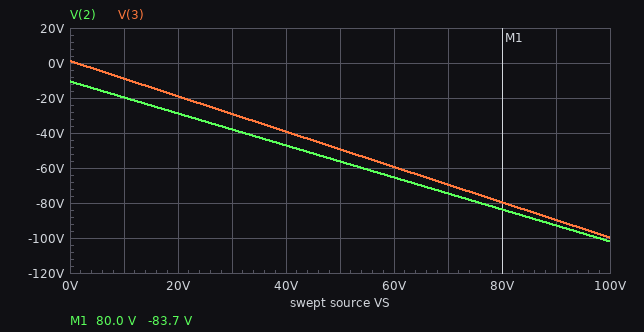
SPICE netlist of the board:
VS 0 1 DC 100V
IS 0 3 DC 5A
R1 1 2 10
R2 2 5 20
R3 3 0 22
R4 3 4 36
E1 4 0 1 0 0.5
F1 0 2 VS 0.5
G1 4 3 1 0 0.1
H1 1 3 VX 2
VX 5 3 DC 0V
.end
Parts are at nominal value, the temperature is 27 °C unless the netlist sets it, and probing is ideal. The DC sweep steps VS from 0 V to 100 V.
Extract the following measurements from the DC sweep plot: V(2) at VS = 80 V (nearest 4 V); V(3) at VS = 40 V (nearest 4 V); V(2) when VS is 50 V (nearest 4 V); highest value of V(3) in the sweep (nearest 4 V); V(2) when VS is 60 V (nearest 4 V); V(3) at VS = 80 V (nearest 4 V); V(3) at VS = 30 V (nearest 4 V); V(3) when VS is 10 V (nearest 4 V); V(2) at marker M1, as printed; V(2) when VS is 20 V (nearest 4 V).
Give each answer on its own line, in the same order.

-84 V
-40 V
-56 V
0 V
-64 V
-80 V
-28 V
-8 V
-83.7 V
-28 V
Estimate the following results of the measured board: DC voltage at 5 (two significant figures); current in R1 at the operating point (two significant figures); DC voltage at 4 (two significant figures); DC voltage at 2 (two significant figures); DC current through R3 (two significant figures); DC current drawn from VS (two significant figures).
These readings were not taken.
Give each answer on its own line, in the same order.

-100 V
200 mA
-50 V
-100 V
4.5 A
610 mA
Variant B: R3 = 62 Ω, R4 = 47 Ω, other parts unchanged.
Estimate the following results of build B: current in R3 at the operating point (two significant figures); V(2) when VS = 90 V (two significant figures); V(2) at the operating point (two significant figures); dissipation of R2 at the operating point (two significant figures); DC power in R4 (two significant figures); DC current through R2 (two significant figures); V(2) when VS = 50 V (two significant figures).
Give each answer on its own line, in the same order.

1.6 A
-87 V
-95 V
1.5 W
54 W
270 mA
-53 V
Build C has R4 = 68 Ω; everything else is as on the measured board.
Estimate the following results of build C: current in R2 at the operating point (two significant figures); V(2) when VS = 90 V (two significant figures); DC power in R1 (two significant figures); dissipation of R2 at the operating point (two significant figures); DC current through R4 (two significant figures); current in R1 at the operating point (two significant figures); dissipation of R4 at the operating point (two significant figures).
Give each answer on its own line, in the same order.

33 mA
-92 V
35 mW
22 mW
730 mA
59 mA
37 W
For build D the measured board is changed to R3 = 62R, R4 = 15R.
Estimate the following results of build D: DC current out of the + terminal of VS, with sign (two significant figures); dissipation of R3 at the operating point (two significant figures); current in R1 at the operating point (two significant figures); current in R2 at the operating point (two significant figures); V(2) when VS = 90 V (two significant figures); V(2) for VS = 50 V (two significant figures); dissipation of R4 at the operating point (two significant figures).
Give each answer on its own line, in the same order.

-35 mA
160 W
11 mA
6.3 mA
-91 V
-55 V
170 W
